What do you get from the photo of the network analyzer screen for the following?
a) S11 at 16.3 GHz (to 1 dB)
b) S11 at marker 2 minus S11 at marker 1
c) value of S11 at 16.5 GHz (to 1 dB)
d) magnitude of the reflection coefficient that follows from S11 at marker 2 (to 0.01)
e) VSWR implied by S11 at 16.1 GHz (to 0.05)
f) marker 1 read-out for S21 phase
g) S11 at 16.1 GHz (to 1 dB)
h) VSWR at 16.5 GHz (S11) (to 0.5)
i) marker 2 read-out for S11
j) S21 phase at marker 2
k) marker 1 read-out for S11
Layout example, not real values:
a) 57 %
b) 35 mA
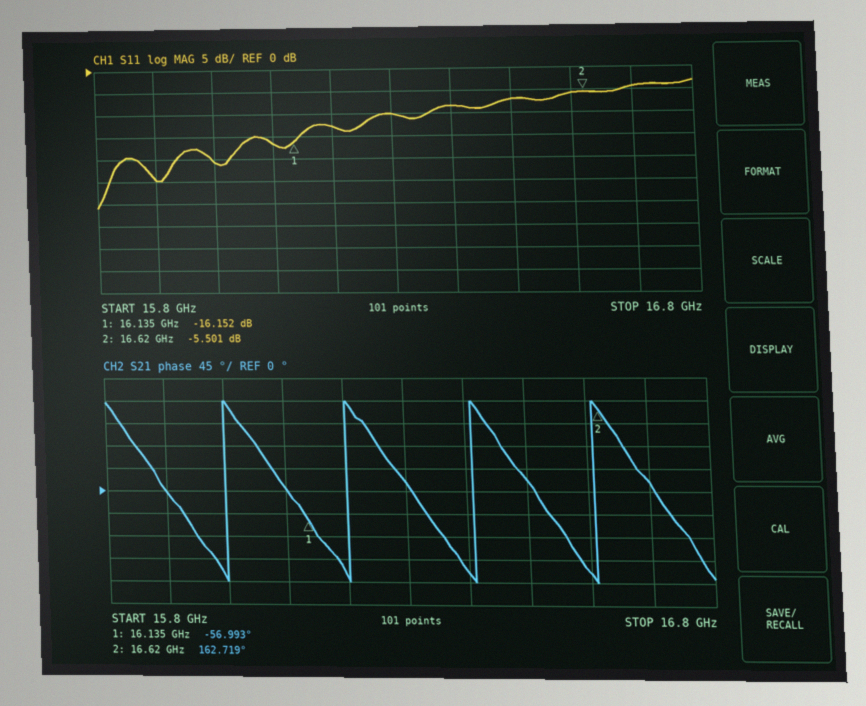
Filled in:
a) -10 dB
b) 10.651 dB
c) -7 dB
d) 0.53
e) 1.35
f) -56.993°
g) -17 dB
h) 2.5
i) -5.501 dB
j) 162.719°
k) -16.152 dB
